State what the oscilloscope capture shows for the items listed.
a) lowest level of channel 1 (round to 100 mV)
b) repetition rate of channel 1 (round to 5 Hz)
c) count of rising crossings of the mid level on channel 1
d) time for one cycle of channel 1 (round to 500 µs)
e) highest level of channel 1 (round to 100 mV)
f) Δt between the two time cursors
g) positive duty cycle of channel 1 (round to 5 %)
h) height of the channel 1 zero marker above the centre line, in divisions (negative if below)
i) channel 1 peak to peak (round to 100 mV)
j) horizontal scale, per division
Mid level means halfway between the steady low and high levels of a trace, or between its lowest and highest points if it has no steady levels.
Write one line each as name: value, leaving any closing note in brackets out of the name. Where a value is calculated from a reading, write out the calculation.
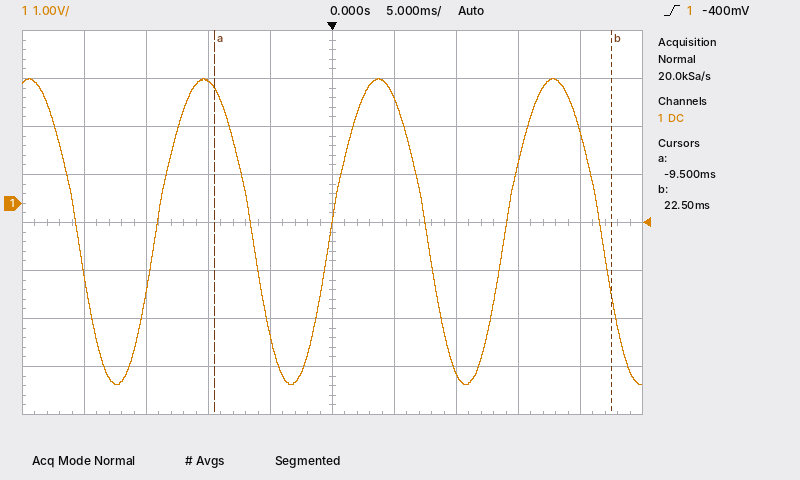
lowest level of channel 1: -3.8 V
repetition rate of channel 1: 1 / 14.0 ms ≈ 71.4 Hz, so 70 Hz to the nearest 5 Hz
count of rising crossings of the mid level on channel 1: 3
time for one cycle of channel 1: 14.0 ms
highest level of channel 1: 2.6 V
Δt between the two time cursors: 22.5 ms − (-9.5 ms) = 32.0 ms
positive duty cycle of channel 1: 55 %
height of the channel 1 zero marker above the centre line, in divisions: +0.4 div
channel 1 peak to peak: 2.6 V − (-3.8 V) = 6.4 V
horizontal scale, per division: 5 ms
